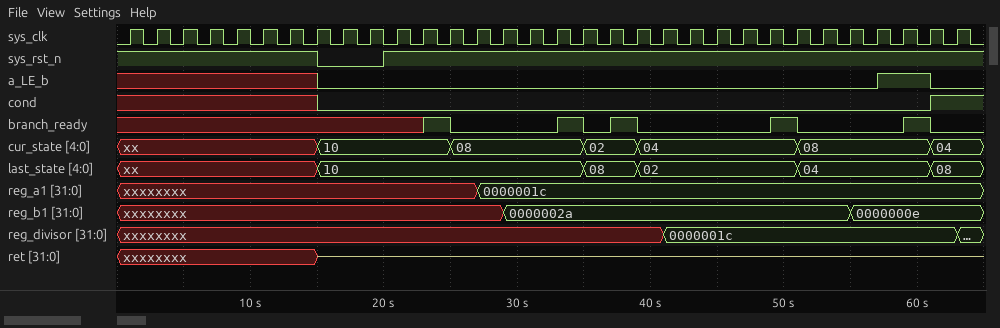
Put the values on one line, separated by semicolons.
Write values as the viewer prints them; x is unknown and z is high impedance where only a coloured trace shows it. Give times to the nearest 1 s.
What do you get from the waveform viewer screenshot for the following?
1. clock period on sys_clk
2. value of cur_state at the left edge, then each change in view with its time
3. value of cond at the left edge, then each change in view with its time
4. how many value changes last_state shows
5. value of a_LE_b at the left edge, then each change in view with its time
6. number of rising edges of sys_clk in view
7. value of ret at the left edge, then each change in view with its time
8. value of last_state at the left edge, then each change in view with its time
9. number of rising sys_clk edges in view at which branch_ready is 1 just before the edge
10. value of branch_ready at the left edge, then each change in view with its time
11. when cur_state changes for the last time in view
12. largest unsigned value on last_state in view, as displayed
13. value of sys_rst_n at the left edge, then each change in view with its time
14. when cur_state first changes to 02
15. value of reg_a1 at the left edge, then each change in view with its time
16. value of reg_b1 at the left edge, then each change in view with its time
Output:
2 s; xx, 10 at 15 s, 08 at 25 s, 02 at 35 s, 04 at 39 s, 08 at 51 s, 04 at 61 s; x, 0 at 15 s, 1 at 61 s; 5; x, 0 at 15 s, 1 at 57 s, 0 at 61 s; 32; xxxxxxxx, z at 15 s; xx, 10 at 15 s, 08 at 35 s, 02 at 39 s, 04 at 51 s, 08 at 61 s; 5; x, 1 at 23 s, 0 at 25 s, 1 at 33 s, 0 at 35 s, 1 at 37 s, 0 at 39 s, 1 at 49 s, 0 at 51 s, 1 at 59 s, 0 at 61 s; 61 s; 10; 1, 0 at 15 s, 1 at 20 s; 35 s; xxxxxxxx, 0000001c at 27 s; xxxxxxxx, 0000002a at 29 s, 0000000e at 55 s
